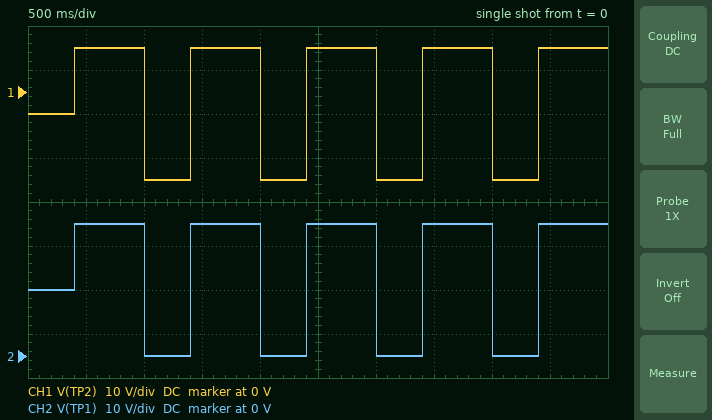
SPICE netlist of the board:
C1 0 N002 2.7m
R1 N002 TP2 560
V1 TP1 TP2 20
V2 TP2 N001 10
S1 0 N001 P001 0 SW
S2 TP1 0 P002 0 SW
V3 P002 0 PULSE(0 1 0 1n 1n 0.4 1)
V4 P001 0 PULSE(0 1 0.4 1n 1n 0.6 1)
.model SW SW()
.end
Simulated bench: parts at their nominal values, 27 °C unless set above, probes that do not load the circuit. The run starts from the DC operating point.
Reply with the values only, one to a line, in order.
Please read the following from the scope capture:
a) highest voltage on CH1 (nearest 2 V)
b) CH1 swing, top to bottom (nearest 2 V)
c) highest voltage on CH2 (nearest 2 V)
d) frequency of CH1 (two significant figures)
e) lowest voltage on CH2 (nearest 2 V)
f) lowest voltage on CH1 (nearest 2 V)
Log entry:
10 V
30 V
30 V
1.0 Hz
0 V
-20 V
